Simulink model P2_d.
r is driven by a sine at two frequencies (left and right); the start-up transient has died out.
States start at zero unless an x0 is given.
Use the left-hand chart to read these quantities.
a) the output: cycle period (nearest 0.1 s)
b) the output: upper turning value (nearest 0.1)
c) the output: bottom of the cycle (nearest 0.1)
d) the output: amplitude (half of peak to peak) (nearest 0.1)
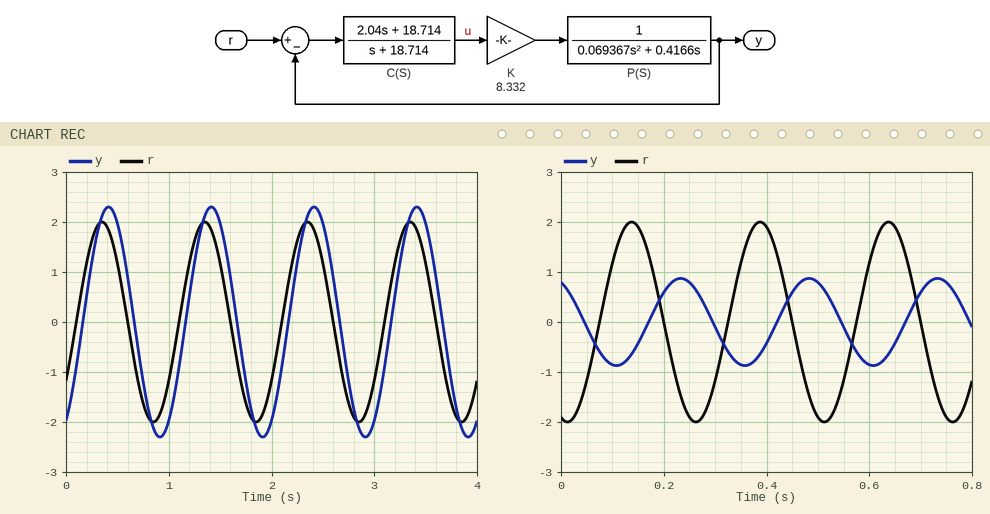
1.0 s
2.3
-2.3
2.3
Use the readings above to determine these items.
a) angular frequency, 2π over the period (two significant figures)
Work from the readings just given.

6.3 rad/s
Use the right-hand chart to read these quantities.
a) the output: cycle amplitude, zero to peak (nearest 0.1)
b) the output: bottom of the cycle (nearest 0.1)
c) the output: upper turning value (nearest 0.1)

0.9
-0.9
0.9
